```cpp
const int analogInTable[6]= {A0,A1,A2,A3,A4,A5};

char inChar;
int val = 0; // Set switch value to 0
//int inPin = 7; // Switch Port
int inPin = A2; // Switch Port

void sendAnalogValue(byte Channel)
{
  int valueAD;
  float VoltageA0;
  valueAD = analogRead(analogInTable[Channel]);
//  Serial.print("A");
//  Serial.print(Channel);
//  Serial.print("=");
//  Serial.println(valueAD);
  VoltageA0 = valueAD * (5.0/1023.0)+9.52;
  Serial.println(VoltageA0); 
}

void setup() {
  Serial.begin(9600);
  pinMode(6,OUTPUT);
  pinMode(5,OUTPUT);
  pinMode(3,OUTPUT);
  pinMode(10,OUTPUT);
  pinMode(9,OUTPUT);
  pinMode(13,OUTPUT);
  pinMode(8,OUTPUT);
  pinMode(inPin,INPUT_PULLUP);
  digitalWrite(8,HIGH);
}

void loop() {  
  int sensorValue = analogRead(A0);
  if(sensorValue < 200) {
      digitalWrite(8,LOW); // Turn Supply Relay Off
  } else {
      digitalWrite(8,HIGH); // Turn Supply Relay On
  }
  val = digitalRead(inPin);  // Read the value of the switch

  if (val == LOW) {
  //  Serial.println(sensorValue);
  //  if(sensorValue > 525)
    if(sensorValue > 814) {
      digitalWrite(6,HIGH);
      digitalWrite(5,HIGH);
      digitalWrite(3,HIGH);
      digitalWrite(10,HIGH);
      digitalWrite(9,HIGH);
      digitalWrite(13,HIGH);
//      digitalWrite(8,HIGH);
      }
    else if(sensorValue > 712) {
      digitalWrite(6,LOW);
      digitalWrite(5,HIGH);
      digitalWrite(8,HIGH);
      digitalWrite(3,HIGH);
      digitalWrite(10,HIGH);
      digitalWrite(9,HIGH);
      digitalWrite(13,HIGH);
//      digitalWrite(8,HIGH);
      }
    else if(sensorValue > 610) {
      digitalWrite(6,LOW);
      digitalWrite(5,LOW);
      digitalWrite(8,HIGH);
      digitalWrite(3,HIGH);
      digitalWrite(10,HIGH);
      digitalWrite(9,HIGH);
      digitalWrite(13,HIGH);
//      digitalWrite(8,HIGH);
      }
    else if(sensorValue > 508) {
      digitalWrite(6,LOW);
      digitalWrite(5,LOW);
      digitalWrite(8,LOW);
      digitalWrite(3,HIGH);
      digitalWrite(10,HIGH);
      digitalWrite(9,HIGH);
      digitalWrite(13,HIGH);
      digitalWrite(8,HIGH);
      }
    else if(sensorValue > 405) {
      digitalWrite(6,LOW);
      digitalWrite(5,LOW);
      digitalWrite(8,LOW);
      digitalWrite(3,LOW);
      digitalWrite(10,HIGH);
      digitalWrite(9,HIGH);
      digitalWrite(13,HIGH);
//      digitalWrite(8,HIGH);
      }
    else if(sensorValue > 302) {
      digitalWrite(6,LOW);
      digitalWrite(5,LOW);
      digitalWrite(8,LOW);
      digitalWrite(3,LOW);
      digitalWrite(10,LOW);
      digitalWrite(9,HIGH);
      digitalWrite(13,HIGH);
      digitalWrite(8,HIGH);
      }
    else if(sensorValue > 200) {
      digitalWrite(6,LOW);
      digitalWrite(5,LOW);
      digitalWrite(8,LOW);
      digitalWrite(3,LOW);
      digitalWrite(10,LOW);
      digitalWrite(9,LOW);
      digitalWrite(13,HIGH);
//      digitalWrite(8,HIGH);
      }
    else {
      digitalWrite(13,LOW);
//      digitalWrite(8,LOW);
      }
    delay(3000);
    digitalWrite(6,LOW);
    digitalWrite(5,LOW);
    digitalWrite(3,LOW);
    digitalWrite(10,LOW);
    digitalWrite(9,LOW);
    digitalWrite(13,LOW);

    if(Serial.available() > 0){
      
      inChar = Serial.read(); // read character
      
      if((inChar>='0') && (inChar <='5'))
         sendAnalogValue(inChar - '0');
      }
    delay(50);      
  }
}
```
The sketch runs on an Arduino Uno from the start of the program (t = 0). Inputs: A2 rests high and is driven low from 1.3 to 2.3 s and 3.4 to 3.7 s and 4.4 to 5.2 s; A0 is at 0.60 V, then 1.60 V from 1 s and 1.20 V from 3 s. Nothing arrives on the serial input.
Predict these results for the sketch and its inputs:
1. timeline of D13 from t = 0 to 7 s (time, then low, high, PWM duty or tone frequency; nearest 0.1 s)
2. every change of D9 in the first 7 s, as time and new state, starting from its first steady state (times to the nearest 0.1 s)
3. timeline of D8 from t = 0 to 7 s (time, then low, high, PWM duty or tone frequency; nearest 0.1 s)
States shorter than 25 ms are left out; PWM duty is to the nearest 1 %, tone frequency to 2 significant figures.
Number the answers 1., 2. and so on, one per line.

1. 0 s low; 1.3 s high; 4.3 s low; 4.4 s high
2. 0 s low; 1.3 s high; 4.3 s low
3. 0 s low; 1 s high; 4.4 s low
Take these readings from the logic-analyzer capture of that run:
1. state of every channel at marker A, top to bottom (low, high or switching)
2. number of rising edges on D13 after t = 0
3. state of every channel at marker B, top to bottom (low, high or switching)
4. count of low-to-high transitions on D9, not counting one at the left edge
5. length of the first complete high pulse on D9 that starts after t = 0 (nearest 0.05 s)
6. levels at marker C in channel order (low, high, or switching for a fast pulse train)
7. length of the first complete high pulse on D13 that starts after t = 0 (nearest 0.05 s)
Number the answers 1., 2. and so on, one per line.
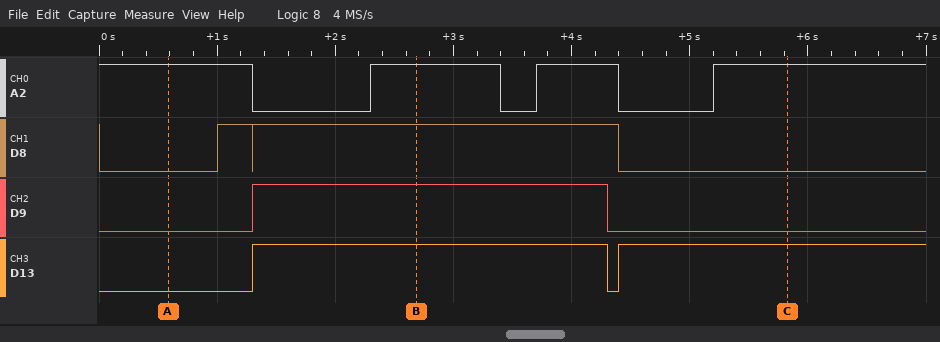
1. A2 high, D8 low, D9 low, D13 low
2. 2
3. A2 high, D8 high, D9 high, D13 high
4. 1
5. 3.00 s
6. A2 high, D8 low, D9 low, D13 high
7. 3.00 s
